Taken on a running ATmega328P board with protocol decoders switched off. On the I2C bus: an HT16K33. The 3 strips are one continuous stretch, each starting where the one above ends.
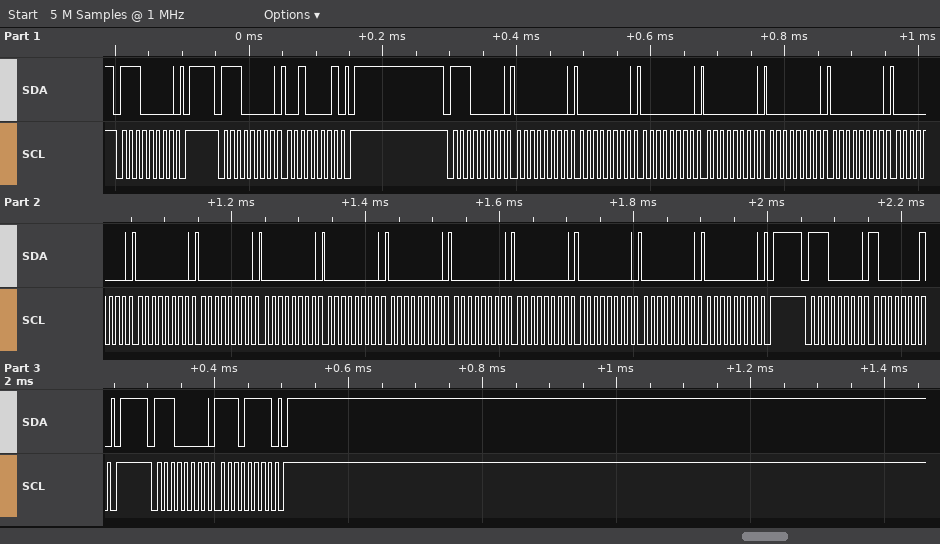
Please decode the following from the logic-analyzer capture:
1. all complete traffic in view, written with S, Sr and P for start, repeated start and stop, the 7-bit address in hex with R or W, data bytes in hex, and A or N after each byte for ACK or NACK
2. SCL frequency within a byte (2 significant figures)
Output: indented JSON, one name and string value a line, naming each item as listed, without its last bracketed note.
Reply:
{
  "all complete traffic in view, written with S, Sr and P for start, repeated start and stop, the 7-bit address in hex with R or W, data bytes in hex, and A or N after each byte for ACK or NACK": "S 70W A P S 70W A 21 A P S 70W A 00 A 00 A 00 A 00 A 00 A 00 A 00 A 00 A 00 A 00 A 00 A 00 A 00 A 00 A 00 A 00 A 00 A P S 70W A 81 A P S 70W A EF A P",
  "SCL frequency within a byte": "100 kHz"
}
